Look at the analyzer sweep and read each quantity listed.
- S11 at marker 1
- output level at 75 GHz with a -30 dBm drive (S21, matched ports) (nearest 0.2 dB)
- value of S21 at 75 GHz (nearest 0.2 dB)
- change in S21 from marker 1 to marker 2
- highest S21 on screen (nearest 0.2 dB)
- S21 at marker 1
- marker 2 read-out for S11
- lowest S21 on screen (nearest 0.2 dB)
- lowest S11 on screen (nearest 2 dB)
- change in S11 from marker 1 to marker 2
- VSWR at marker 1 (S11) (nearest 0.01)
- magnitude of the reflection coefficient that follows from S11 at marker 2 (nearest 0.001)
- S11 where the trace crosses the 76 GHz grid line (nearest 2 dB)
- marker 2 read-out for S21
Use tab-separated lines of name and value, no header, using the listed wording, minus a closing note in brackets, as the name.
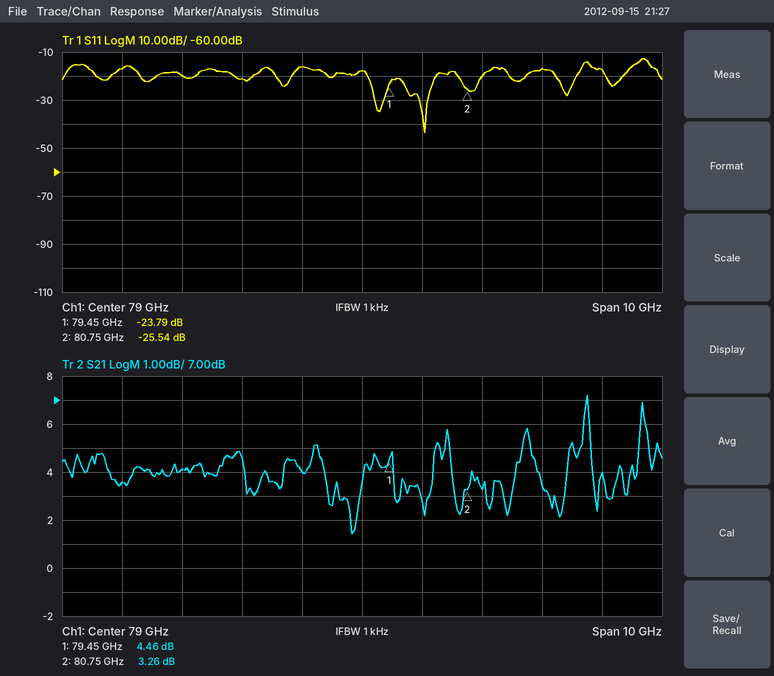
S11 at marker 1	-23.79 dB
output level at 75 GHz with a -30 dBm drive (S21, matched ports)	-26.4 dBm
value of S21 at 75 GHz	3.6 dB
change in S21 from marker 1 to marker 2	-1.20 dB
highest S21 on screen	7.2 dB
S21 at marker 1	4.46 dB
marker 2 read-out for S11	-25.54 dB
lowest S21 on screen	1.4 dB
lowest S11 on screen	-44 dB
change in S11 from marker 1 to marker 2	-1.75 dB
VSWR at marker 1 (S11)	1.14
magnitude of the reflection coefficient that follows from S11 at marker 2	0.053
S11 where the trace crosses the 76 GHz grid line	-20 dB
marker 2 read-out for S21	3.26 dB
